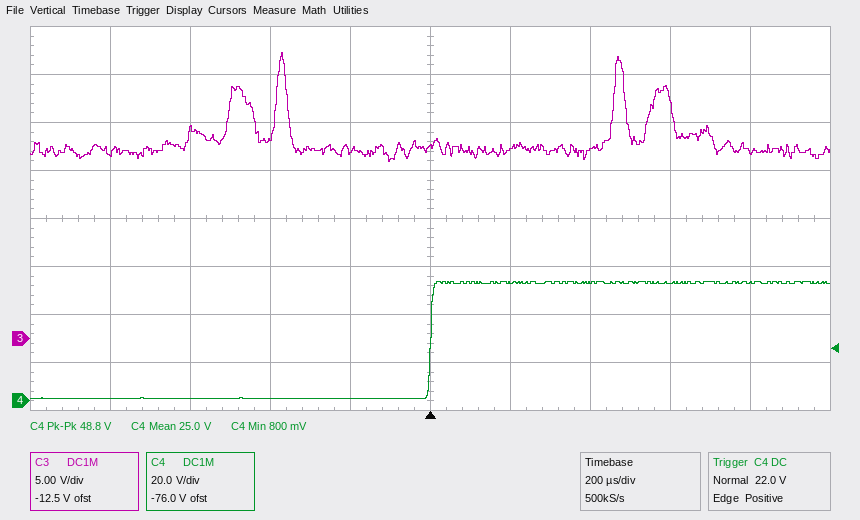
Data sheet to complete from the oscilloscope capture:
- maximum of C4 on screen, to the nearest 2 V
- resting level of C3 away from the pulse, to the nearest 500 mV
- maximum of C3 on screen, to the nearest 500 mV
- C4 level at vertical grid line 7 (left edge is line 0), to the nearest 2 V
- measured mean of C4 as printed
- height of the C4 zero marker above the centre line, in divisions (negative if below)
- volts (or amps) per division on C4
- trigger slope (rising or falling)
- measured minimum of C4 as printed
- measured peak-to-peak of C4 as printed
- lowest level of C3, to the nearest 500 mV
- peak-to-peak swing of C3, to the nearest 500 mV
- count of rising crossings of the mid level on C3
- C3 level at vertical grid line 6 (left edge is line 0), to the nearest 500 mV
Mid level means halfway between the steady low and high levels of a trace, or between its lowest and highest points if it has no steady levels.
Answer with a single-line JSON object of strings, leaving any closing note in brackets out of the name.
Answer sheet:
{"maximum of C4 on screen, to the nearest 2 V": "50 V", "resting level of C3 away from the pulse, to the nearest 500 mV": "19.5 V", "maximum of C3 on screen, to the nearest 500 mV": "30.0 V", "C4 level at vertical grid line 7 (left edge is line 0), to the nearest 2 V": "50 V", "measured mean of C4 as printed": "25.0 V", "height of the C4 zero marker above the centre line, in divisions": "-3.8 div", "volts (or amps) per division on C4": "20 V", "trigger slope": "rising", "measured minimum of C4 as printed": "800 mV", "measured peak-to-peak of C4 as printed": "48.8 V", "lowest level of C3, to the nearest 500 mV": "18.5 V", "peak-to-peak swing of C3, to the nearest 500 mV": "11.5 V", "count of rising crossings of the mid level on C3": "4", "C3 level at vertical grid line 6 (left edge is line 0), to the nearest 500 mV": "20.0 V"}
